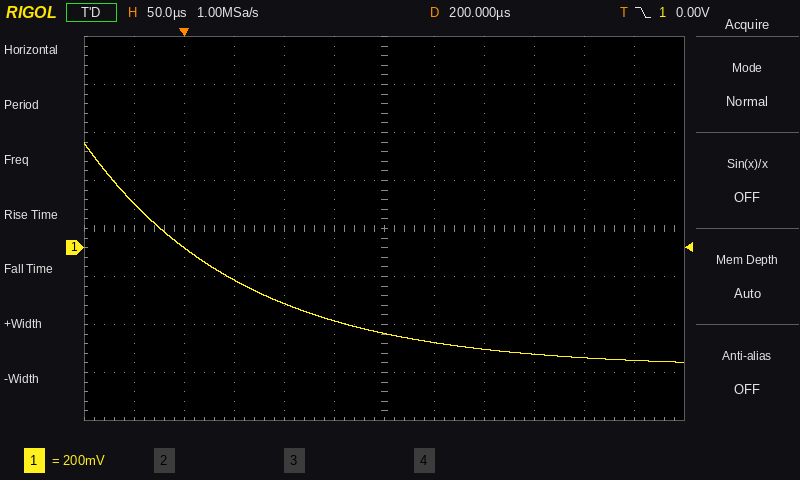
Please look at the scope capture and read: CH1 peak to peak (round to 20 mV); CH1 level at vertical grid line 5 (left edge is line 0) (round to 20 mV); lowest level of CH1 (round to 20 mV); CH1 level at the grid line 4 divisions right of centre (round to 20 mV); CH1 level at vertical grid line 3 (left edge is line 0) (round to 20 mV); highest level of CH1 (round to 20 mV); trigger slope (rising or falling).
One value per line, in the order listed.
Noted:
920 mV
-300 mV
-480 mV
-460 mV
-140 mV
440 mV
falling
